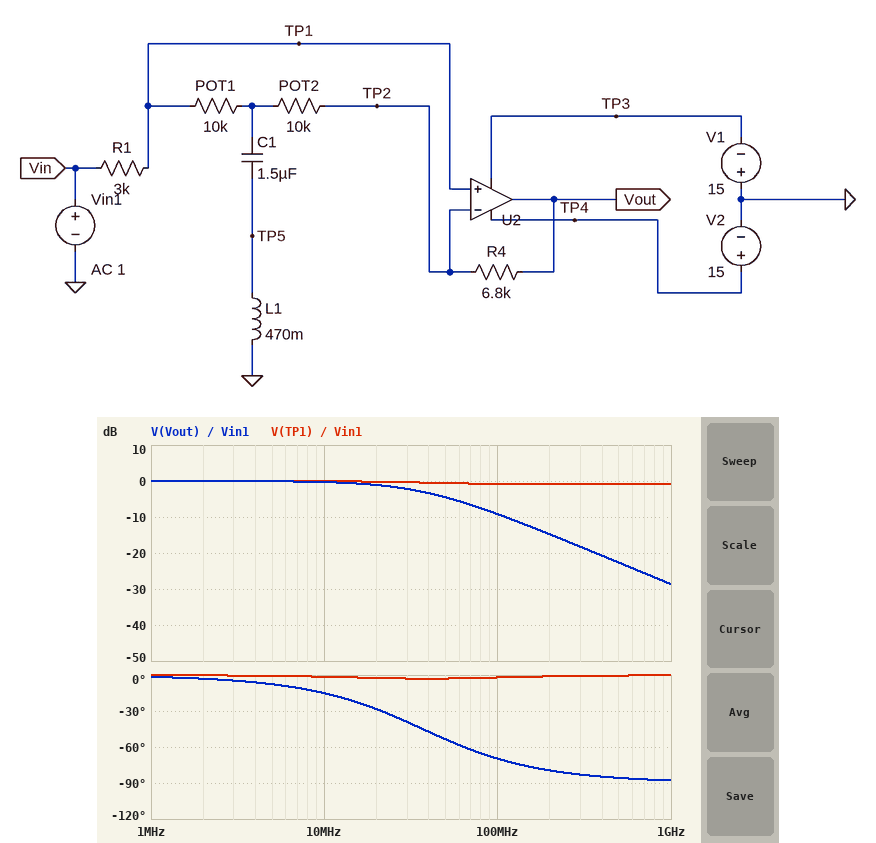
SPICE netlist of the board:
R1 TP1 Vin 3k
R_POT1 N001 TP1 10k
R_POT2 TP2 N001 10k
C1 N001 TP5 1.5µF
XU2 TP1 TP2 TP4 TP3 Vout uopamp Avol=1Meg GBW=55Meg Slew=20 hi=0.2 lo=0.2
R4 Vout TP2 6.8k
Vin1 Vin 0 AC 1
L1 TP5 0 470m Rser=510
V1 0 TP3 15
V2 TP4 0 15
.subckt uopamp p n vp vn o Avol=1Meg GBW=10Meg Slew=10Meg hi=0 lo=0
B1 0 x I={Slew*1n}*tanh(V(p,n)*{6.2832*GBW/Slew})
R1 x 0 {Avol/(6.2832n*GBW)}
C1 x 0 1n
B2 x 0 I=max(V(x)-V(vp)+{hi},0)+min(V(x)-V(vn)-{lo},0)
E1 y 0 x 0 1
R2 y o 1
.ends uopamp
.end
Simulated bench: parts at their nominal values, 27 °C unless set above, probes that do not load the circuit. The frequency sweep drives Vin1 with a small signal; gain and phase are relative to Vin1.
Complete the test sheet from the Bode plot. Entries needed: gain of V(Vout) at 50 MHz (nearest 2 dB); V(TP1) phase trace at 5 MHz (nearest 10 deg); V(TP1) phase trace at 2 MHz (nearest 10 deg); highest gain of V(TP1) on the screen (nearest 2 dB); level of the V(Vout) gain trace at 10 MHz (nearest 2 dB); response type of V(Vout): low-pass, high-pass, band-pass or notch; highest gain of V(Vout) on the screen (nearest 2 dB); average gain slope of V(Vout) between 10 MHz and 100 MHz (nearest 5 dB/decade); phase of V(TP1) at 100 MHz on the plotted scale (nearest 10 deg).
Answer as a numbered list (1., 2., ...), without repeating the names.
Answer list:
1. -4 dB
2. 0 deg
3. 0 deg
4. 0 dB
5. 0 dB
6. low-pass
7. 0 dB
8. -10 dB/decade
9. 0 deg
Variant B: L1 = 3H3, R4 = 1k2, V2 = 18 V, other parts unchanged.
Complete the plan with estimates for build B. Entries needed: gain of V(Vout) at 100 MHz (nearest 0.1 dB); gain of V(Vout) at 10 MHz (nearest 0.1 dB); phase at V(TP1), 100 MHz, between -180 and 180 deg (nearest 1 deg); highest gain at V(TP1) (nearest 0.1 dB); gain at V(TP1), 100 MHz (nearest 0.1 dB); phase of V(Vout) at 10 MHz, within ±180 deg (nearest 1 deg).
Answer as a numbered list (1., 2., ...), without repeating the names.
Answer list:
1. -7.7 dB
2. -0.2 dB
3. -3 deg
4. 0 dB
5. -0.9 dB
6. -12 deg
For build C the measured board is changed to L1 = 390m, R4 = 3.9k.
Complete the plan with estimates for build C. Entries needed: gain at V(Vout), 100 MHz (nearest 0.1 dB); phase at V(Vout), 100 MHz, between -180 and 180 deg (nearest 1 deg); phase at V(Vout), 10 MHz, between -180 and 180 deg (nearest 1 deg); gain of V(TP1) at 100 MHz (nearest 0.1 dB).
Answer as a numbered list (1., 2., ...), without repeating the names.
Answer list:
1. -8.4 dB
2. -68 deg
3. -14 deg
4. -0.9 dB
